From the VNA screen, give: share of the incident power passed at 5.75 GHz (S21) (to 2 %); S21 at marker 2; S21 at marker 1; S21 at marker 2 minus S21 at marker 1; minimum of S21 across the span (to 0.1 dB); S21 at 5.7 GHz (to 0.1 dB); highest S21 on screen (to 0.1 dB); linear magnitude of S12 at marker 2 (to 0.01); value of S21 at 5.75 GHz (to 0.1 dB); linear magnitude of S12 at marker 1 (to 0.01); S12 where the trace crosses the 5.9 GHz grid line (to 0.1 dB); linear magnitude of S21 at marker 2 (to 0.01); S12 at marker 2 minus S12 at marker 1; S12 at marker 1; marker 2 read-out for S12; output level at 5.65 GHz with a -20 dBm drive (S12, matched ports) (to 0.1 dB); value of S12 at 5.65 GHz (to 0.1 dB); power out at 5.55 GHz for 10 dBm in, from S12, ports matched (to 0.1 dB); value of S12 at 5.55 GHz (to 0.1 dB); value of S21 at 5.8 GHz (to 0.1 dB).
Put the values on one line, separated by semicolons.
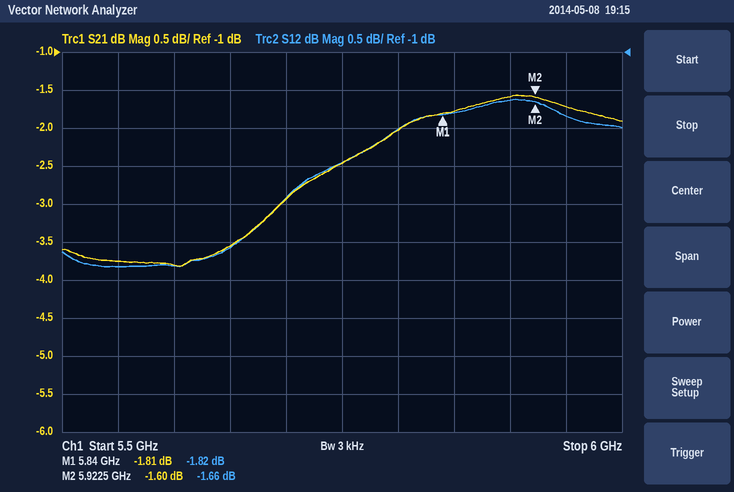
56 %; -1.60 dB; -1.81 dB; 0.21 dB; -3.8 dB; -2.9 dB; -1.6 dB; 0.83; -2.5 dB; 0.81; -1.6 dB; 0.83; 0.16 dB; -1.82 dB; -1.66 dB; -23.6 dBm; -3.6 dB; 6.2 dBm; -3.8 dB; -2.0 dB
